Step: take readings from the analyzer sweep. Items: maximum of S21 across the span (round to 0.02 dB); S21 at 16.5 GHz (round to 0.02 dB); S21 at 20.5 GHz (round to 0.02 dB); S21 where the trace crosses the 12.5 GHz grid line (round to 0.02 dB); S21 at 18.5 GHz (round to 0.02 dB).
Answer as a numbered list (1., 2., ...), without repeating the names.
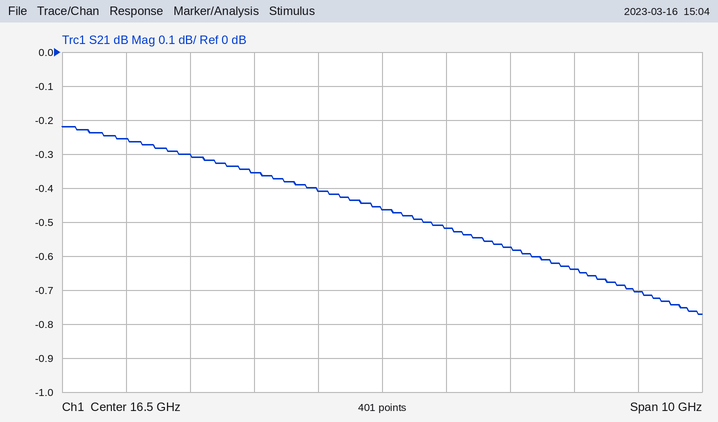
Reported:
1. -0.22 dB
2. -0.46 dB
3. -0.70 dB
4. -0.26 dB
5. -0.58 dB
